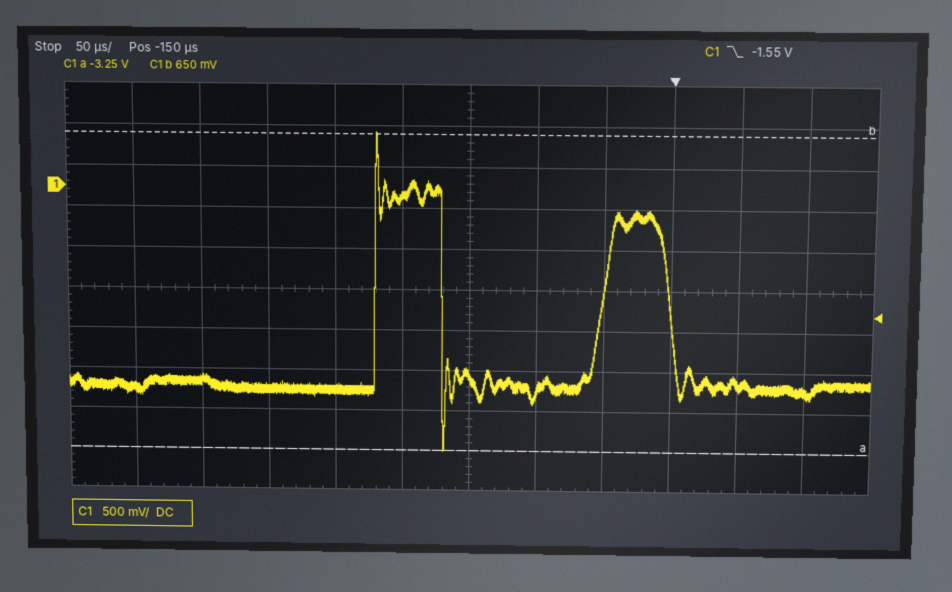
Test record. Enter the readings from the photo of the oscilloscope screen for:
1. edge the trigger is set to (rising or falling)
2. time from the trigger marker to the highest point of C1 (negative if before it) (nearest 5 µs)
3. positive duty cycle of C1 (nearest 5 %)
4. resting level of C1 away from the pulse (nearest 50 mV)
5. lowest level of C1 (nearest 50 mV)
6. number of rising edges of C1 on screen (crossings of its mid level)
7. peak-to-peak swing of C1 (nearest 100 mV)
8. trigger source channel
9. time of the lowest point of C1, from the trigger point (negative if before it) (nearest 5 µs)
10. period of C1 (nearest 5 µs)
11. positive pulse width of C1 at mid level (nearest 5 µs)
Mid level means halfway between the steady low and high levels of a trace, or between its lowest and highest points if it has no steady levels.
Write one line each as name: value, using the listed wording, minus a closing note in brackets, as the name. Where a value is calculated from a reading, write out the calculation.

edge the trigger is set to: falling
time from the trigger marker to the highest point of C1 (negative if before it): -220 µs
positive duty cycle of C1: 50 µs / 170 µs ≈ 29.4 %, so 30 % to the nearest 5 %
resting level of C1 away from the pulse: -2.45 V
lowest level of C1: -3.25 V
number of rising edges of C1 on screen: 2
peak-to-peak swing of C1: 3.90 V
trigger source channel: C1
time of the lowest point of C1, from the trigger point (negative if before it): -170 µs
period of C1: 170 µs
positive pulse width of C1 at mid level: 50 µs
